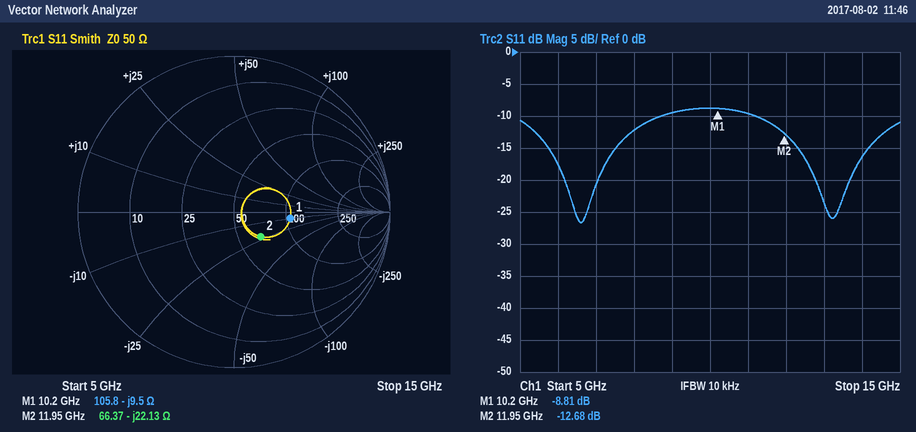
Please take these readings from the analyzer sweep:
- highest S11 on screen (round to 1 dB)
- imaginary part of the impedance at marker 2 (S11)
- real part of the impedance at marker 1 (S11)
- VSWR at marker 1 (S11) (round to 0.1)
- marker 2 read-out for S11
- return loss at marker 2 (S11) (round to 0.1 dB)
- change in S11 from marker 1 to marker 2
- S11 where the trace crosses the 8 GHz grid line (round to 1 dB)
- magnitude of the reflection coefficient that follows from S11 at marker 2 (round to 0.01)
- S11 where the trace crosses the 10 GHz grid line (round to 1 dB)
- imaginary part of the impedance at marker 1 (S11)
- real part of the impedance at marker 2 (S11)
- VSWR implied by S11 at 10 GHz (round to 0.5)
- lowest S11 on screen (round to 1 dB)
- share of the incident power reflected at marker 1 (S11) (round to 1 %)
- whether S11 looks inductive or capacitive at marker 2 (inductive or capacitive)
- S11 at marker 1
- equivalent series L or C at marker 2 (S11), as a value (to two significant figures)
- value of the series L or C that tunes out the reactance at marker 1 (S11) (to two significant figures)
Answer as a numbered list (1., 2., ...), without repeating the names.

1. -9 dB
2. -22.13 Ω
3. 105.8 Ω
4. 2.1
5. -12.68 dB
6. 12.7 dB
7. -3.87 dB
8. -12 dB
9. 0.23
10. -9 dB
11. -9.5 Ω
12. 66.37 Ω
13. 2.0
14. -27 dB
15. 13 %
16. capacitive
17. -8.81 dB
18. 600 fF
19. 150 pH
